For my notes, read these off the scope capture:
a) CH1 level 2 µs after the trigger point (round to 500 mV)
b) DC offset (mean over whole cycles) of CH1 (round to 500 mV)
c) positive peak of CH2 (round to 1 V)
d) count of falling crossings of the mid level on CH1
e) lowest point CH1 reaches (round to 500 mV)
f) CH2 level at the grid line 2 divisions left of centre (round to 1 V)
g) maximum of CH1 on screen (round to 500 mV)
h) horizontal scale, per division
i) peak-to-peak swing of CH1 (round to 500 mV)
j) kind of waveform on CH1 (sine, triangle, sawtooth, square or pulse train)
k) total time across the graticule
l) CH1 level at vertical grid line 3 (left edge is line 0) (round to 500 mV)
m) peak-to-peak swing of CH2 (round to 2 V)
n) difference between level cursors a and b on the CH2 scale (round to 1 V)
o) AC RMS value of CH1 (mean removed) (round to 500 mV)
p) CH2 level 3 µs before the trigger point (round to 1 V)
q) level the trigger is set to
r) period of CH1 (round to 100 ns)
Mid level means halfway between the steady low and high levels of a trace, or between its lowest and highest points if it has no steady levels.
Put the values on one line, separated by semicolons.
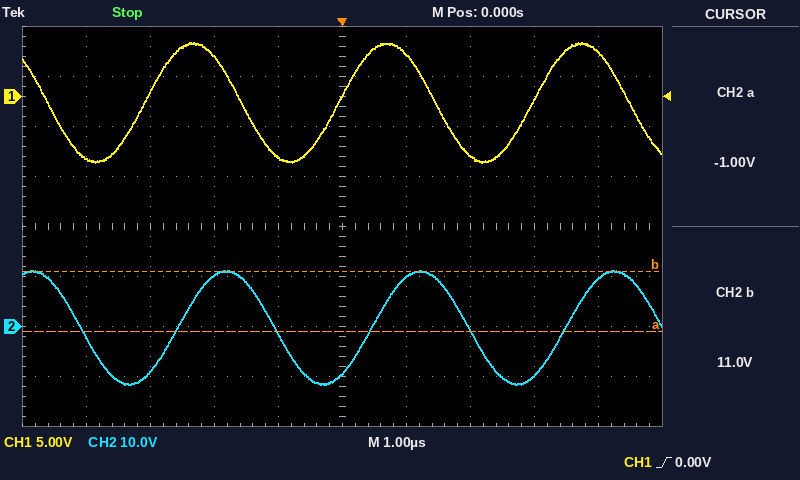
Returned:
-6.0 V; -500 mV; 11 V; 4; -6.5 V; 10 V; 5.5 V; 1 µs; 12.0 V; sine; 10 µs; 4.0 V; 22 V; 12 V; 4.0 V; -9 V; 0.00 V; 3.0 µs
